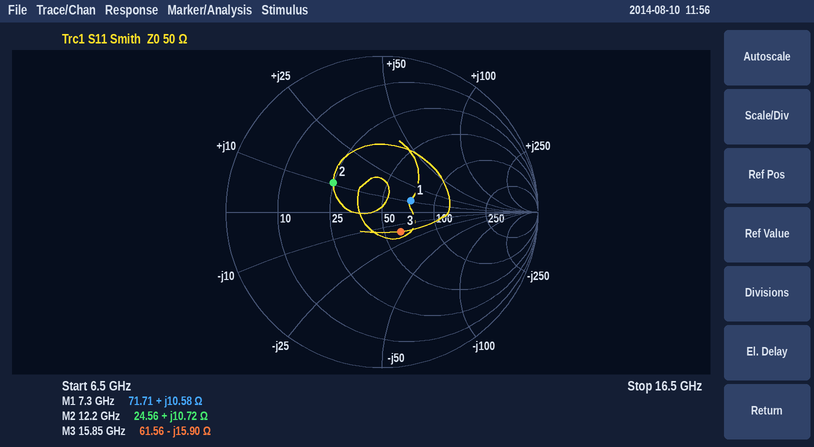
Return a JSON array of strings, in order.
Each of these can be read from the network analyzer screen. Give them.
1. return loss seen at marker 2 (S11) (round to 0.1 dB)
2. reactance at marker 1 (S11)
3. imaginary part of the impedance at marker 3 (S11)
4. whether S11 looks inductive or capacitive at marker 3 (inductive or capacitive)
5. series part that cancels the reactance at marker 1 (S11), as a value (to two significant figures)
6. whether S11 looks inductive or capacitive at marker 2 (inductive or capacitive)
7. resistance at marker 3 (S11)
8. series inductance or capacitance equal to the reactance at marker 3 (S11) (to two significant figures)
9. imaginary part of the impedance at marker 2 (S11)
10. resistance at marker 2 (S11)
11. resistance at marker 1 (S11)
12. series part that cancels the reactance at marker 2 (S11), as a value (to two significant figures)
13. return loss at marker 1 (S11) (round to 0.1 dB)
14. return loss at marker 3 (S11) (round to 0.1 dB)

["8.7 dB", "+10.58 Ω", "-15.90 Ω", "capacitive", "2.1 pF", "inductive", "61.56 Ω", "630 fF", "+10.72 Ω", "24.56 Ω", "71.71 Ω", "1.2 pF", "14.1 dB", "15.2 dB"]
